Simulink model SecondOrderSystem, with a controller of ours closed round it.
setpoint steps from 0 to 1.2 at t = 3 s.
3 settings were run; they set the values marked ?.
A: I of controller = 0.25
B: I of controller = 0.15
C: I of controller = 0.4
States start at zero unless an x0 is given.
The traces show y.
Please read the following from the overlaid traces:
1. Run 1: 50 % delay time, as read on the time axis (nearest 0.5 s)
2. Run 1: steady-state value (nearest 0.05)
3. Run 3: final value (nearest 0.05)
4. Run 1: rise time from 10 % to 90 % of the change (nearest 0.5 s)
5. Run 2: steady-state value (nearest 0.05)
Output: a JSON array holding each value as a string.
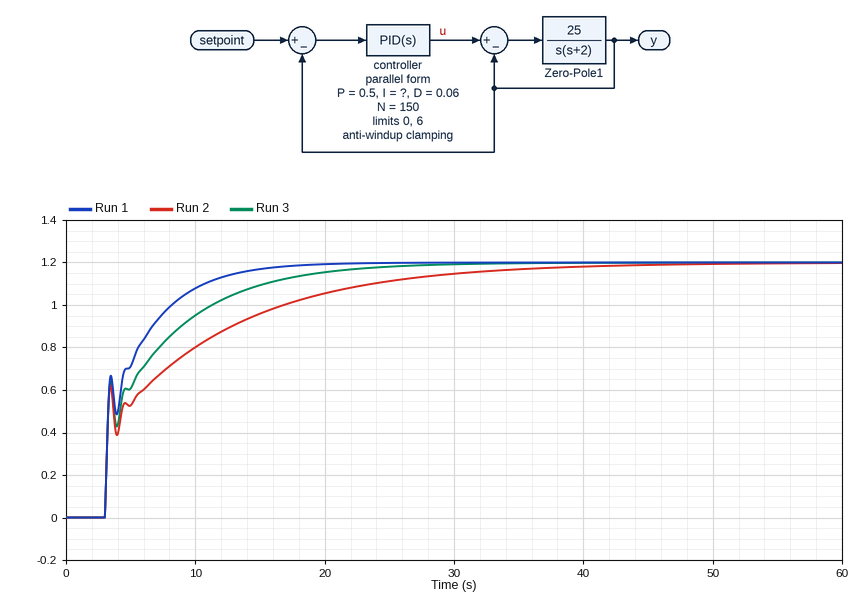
["3.5 s", "1.20", "1.20", "7.0 s", "1.20"]
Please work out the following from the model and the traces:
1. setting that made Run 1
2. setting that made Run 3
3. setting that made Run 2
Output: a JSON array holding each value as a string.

["C", "A", "B"]
